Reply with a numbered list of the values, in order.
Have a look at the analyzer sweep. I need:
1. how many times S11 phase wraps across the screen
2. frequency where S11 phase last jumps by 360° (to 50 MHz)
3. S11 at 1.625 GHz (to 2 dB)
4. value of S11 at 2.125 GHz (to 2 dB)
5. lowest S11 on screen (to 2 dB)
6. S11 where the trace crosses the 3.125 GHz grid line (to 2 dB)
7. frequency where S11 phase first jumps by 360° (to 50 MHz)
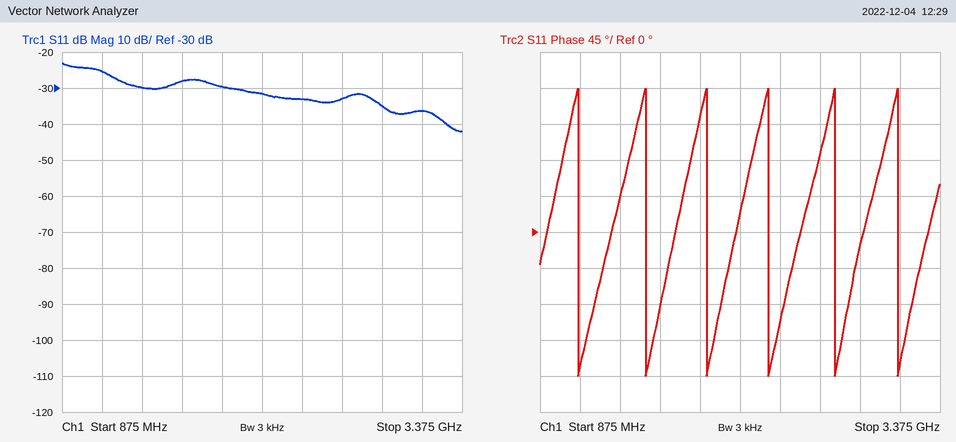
1. 6
2. 3.10 GHz
3. -28 dB
4. -32 dB
5. -42 dB
6. -36 dB
7. 1.10 GHz
